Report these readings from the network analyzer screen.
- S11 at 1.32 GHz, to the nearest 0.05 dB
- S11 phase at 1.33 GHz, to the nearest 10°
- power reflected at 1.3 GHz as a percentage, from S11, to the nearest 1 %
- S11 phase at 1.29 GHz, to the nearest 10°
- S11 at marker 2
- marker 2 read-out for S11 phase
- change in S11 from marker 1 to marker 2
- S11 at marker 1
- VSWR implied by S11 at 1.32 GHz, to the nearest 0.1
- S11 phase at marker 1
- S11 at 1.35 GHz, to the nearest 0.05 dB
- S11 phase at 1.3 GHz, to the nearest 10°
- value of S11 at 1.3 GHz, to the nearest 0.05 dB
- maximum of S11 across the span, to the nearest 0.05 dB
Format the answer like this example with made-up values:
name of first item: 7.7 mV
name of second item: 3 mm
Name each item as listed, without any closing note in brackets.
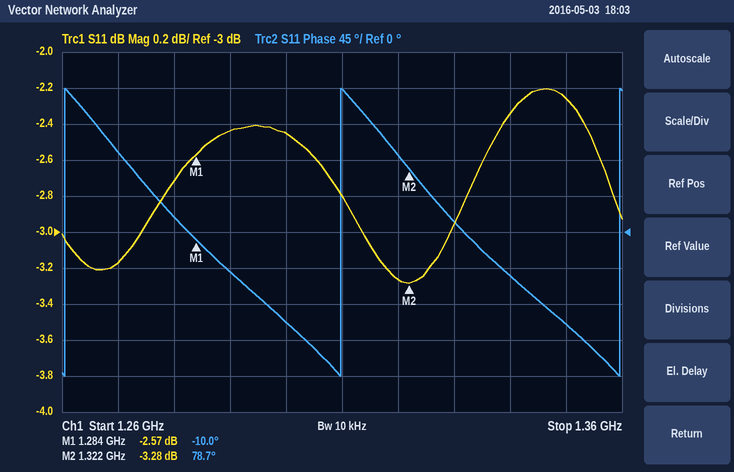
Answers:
S11 at 1.32 GHz, to the nearest 0.05 dB: -3.25 dB
S11 phase at 1.33 GHz, to the nearest 10°: 10°
power reflected at 1.3 GHz as a percentage, from S11, to the nearest 1 %: 57 %
S11 phase at 1.29 GHz, to the nearest 10°: -50°
S11 at marker 2: -3.28 dB
marker 2 read-out for S11 phase: 78.7°
change in S11 from marker 1 to marker 2: -0.71 dB
S11 at marker 1: -2.57 dB
VSWR implied by S11 at 1.32 GHz, to the nearest 0.1: 5.4
S11 phase at marker 1: -10.0°
S11 at 1.35 GHz, to the nearest 0.05 dB: -2.25 dB
S11 phase at 1.3 GHz, to the nearest 10°: -110°
value of S11 at 1.3 GHz, to the nearest 0.05 dB: -2.45 dB
maximum of S11 across the span, to the nearest 0.05 dB: -2.20 dB
